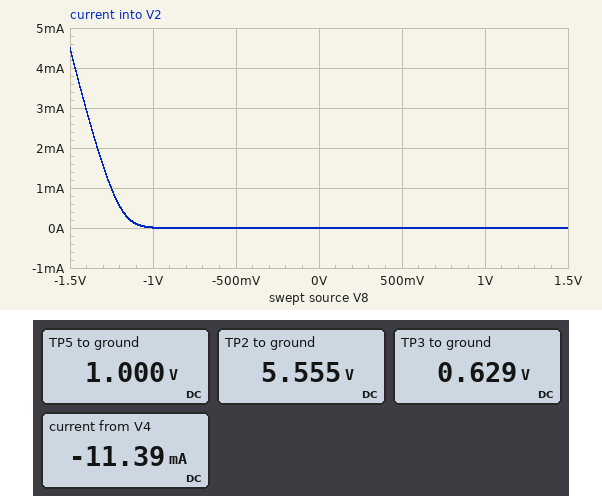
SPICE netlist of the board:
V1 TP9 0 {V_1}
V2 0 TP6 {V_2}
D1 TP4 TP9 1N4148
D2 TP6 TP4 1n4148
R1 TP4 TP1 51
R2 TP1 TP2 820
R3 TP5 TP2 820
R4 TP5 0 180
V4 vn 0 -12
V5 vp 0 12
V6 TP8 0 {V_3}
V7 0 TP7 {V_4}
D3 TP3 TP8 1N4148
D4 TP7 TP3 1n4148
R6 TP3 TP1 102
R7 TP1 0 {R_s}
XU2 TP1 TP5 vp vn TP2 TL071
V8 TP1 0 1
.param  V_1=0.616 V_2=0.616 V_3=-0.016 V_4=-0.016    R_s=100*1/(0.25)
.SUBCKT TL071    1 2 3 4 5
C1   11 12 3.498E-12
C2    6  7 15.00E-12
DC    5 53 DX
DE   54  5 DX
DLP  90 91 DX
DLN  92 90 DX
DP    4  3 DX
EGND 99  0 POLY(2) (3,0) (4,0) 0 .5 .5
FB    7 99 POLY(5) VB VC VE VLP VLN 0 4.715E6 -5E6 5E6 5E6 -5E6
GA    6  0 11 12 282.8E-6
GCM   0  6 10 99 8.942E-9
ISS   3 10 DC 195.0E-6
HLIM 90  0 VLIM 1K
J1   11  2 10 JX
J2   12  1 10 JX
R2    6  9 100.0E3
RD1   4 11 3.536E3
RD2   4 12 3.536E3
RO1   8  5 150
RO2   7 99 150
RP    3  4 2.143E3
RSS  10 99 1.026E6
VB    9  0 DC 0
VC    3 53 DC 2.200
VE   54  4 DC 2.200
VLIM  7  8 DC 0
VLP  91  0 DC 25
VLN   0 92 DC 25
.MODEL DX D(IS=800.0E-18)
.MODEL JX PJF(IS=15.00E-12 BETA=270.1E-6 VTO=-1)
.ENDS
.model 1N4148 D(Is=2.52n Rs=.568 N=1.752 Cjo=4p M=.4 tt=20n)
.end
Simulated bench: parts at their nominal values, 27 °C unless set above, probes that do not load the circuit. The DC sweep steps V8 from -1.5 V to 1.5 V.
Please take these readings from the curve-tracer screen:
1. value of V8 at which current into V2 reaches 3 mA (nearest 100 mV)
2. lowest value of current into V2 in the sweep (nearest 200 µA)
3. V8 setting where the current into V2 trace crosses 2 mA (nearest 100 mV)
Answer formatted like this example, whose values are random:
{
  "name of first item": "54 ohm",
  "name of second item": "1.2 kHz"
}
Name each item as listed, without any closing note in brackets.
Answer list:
{
  "value of V8 at which current into V2 reaches 3 mA": "-1.4 V",
  "lowest value of current into V2 in the sweep": "0 A",
  "V8 setting where the current into V2 trace crosses 2 mA": "-1.3 V"
}
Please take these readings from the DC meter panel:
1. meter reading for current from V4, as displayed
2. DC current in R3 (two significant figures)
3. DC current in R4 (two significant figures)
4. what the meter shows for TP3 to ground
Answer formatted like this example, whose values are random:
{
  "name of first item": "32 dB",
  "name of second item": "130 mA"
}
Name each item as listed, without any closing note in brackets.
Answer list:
{
  "meter reading for current from V4, as displayed": "-11.39 mA",
  "DC current in R3": "5.6 mA",
  "DC current in R4": "5.6 mA",
  "what the meter shows for TP3 to ground": "0.629 V"
}
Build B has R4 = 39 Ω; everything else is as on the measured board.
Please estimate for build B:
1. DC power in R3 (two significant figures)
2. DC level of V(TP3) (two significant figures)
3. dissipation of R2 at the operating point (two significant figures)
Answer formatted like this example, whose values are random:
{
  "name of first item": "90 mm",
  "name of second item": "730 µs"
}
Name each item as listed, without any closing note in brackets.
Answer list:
{
  "DC power in R3": "120 mW",
  "DC level of V(TP3)": "630 mV",
  "dissipation of R2 at the operating point": "110 mW"
}
